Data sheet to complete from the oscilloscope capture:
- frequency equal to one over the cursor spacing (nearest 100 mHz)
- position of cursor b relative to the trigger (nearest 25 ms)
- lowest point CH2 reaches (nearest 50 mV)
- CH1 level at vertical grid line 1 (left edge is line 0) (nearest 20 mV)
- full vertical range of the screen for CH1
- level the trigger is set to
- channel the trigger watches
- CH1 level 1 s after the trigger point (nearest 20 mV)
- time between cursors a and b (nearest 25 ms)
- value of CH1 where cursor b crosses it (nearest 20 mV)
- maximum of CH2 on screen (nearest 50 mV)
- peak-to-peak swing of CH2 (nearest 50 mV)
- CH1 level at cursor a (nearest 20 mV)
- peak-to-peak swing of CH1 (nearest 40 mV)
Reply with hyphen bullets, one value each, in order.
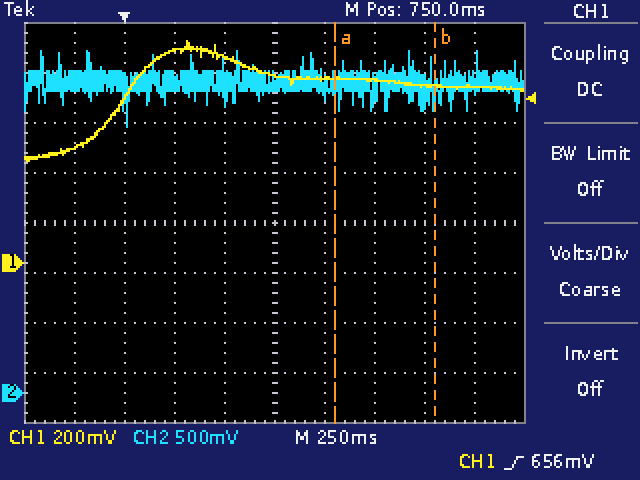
- 2.0 Hz
- +1.550 s
- 2.65 V
- 460 mV
- 1.6 V
- 656 mV
- CH1
- 740 mV
- 500 ms
- 700 mV
- 3.40 V
- 750 mV
- 740 mV
- 480 mV
